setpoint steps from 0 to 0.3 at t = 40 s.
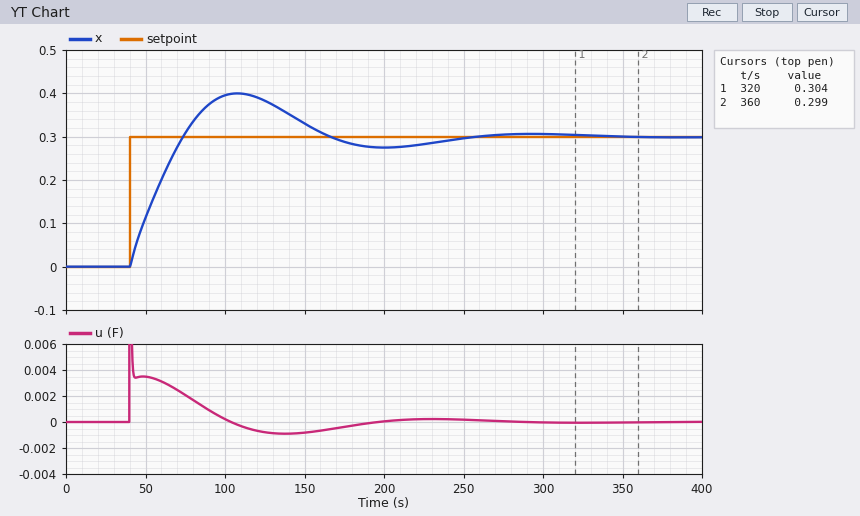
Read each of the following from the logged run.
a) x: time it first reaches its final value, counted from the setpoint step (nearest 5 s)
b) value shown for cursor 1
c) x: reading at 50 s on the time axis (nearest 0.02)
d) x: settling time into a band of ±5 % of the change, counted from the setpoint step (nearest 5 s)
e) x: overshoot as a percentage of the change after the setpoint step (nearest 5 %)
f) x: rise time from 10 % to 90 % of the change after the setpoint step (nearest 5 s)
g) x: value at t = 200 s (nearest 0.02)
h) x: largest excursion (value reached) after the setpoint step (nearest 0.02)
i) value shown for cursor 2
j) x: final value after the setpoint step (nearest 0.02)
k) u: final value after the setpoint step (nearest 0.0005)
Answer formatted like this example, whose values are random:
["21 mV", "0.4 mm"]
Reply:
["35 s", "0.304", "0.12", "190 s", "35 %", "25 s", "0.28", "0.40", "0.299", "0.30", "0.0000"]
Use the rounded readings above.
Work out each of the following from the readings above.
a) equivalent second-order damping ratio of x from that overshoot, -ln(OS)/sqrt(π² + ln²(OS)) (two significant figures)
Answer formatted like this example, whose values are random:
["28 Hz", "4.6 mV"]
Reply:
["0.32"]
